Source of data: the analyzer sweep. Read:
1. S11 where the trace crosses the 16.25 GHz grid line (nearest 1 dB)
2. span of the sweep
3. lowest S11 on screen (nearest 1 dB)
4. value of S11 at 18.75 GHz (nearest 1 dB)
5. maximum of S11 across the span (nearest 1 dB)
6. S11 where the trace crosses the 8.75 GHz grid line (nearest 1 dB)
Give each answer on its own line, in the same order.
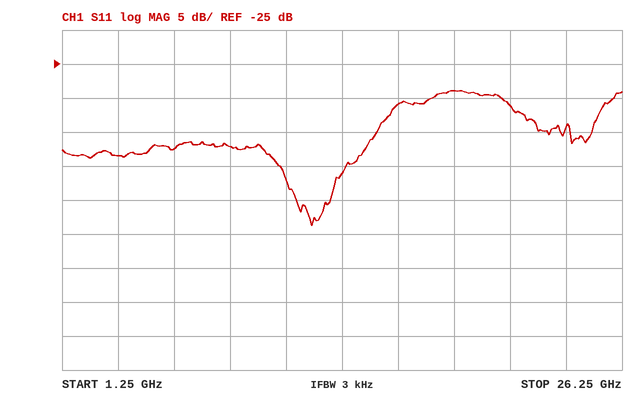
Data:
-31 dB
25 GHz
-49 dB
-29 dB
-29 dB
-37 dB
